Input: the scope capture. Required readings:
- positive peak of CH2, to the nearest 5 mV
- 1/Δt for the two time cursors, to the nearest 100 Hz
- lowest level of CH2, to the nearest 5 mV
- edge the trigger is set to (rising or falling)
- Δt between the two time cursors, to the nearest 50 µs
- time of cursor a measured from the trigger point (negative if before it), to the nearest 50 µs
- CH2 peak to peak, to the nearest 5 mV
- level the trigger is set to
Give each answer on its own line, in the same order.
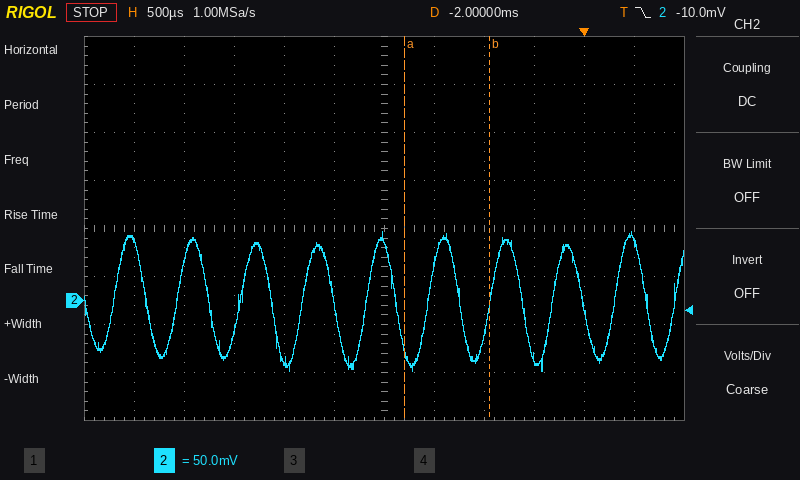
70 mV
1.2 kHz
-75 mV
falling
850 µs
-1.80 ms
145 mV
-10.0 mV
